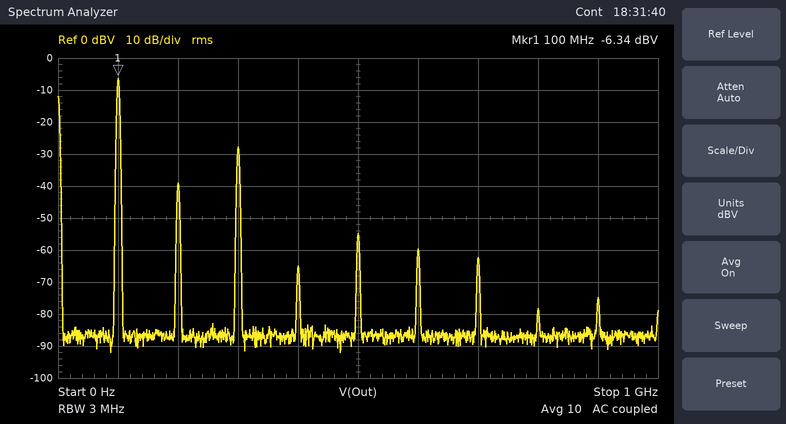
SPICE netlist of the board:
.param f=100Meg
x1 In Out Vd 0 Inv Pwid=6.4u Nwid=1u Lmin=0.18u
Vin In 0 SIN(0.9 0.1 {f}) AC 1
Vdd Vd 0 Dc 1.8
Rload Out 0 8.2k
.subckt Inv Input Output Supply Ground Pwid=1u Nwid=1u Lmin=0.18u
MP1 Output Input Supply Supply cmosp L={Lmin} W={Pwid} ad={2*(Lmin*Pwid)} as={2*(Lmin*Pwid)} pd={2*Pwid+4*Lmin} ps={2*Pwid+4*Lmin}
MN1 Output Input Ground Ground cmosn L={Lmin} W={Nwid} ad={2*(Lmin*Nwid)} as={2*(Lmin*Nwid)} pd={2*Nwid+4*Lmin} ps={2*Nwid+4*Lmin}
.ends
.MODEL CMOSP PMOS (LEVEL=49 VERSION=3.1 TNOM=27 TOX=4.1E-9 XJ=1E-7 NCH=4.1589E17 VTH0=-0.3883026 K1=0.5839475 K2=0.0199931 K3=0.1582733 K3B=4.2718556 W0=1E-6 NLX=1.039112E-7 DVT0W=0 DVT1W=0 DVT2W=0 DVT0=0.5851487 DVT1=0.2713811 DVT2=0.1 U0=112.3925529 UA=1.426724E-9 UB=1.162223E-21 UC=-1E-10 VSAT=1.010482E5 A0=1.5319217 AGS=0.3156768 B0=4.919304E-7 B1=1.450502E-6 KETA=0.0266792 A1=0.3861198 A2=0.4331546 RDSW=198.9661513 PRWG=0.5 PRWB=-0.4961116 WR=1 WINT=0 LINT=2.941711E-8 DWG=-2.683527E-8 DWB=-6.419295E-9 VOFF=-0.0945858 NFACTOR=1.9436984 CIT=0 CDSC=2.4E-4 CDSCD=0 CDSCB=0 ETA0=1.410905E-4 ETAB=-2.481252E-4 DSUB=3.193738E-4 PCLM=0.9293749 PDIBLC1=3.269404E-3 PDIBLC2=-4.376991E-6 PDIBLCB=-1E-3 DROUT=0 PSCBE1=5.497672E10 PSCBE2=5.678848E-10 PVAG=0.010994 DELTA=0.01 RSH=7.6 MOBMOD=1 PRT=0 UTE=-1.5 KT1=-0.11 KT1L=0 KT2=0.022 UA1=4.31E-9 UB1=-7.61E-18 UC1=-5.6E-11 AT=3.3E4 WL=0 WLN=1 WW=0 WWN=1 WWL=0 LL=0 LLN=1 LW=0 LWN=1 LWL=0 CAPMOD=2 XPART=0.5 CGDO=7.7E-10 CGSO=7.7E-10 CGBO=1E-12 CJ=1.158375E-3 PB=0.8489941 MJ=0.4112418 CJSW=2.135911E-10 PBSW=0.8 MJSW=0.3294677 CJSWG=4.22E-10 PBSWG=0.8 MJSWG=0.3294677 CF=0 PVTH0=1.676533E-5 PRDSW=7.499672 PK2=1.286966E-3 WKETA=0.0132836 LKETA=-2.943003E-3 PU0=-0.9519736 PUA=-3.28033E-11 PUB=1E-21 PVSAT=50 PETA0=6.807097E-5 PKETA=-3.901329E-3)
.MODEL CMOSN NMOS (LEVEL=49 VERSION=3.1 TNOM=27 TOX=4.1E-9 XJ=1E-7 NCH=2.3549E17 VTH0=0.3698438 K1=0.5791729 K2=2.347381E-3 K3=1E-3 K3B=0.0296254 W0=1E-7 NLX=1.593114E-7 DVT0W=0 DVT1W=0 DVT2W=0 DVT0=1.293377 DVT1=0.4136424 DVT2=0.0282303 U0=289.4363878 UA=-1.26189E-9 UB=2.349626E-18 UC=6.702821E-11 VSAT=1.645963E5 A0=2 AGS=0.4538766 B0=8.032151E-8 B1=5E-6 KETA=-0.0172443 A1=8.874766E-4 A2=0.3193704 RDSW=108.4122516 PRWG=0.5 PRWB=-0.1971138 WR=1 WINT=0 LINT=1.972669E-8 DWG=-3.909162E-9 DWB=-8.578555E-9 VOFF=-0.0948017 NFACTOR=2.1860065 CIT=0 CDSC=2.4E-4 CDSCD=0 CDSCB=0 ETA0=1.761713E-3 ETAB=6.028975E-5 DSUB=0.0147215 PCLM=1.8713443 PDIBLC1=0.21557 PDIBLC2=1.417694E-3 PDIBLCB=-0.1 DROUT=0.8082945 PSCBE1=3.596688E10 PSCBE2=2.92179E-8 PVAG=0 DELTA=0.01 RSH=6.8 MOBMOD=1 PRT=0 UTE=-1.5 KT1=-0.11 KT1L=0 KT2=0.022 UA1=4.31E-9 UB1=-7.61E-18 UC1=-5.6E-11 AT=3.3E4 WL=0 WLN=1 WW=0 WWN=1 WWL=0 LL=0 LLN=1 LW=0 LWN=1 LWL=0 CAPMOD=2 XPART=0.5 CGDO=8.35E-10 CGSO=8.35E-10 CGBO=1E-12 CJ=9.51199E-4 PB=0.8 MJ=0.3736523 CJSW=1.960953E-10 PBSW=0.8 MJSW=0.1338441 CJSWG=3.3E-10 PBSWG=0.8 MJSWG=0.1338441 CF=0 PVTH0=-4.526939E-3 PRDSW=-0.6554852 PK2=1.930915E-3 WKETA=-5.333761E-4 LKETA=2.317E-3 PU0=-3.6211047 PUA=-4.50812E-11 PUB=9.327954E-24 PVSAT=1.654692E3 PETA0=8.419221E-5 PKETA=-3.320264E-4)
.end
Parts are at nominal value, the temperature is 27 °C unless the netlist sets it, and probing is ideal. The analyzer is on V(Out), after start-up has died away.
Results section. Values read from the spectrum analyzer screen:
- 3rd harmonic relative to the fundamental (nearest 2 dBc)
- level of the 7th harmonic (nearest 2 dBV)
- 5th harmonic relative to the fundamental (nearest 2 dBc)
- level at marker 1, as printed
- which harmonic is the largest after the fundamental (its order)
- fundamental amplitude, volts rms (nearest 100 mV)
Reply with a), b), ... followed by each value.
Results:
a) -22 dBc
b) -62 dBV
c) -48 dBc
d) -6.34 dBV
e) 3
f) 500 mV
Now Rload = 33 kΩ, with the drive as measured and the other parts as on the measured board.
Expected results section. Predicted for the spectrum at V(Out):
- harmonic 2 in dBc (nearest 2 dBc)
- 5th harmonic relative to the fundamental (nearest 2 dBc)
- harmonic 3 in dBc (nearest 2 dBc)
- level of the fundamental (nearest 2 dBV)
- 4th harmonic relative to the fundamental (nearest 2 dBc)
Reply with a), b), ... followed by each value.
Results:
a) -10 dBc
b) -28 dBc
c) -28 dBc
d) -6 dBV
e) -20 dBc
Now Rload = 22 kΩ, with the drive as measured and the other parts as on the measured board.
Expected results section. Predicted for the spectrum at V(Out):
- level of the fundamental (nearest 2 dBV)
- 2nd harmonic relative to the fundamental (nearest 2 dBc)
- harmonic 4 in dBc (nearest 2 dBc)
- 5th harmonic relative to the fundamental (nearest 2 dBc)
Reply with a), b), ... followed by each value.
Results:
a) -6 dBV
b) -12 dBc
c) -22 dBc
d) -42 dBc
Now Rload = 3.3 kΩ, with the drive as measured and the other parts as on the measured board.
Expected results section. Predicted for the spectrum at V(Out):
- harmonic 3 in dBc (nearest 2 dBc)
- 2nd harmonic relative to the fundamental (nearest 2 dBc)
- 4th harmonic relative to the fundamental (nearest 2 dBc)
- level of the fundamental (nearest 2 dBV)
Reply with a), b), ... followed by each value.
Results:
a) -32 dBc
b) -18 dBc
c) -48 dBc
d) -12 dBV
